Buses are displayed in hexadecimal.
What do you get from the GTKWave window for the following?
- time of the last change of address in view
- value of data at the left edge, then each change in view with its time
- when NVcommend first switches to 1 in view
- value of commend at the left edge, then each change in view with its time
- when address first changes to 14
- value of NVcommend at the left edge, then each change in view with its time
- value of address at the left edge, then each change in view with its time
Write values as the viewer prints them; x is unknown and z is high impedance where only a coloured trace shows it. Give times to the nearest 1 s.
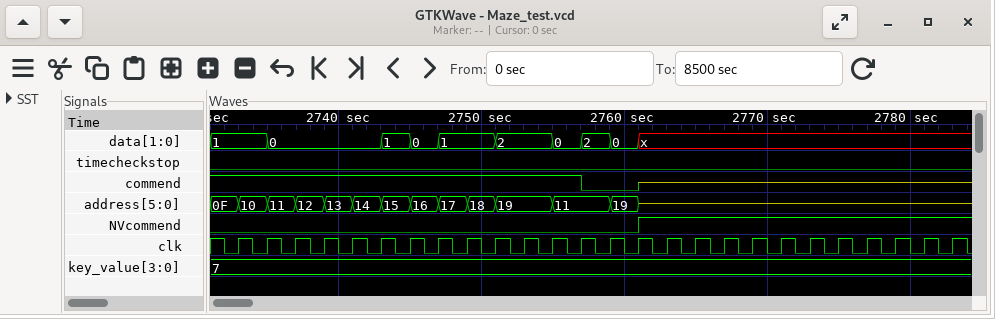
2761 s
1, 0 at 2735 s, 1 at 2743 s, 0 at 2745 s, 1 at 2747 s, 2 at 2751 s, 0 at 2755 s, 2 at 2757 s, 0 at 2759 s, x at 2761 s
2761 s
1, 0 at 2757 s, z at 2761 s
2741 s
0, 1 at 2761 s
0F, 10 at 2733 s, 11 at 2735 s, 12 at 2737 s, 13 at 2739 s, 14 at 2741 s, 15 at 2743 s, 16 at 2745 s, 17 at 2747 s, 18 at 2749 s, 19 at 2751 s, 11 at 2755 s, 19 at 2759 s, z at 2761 s
